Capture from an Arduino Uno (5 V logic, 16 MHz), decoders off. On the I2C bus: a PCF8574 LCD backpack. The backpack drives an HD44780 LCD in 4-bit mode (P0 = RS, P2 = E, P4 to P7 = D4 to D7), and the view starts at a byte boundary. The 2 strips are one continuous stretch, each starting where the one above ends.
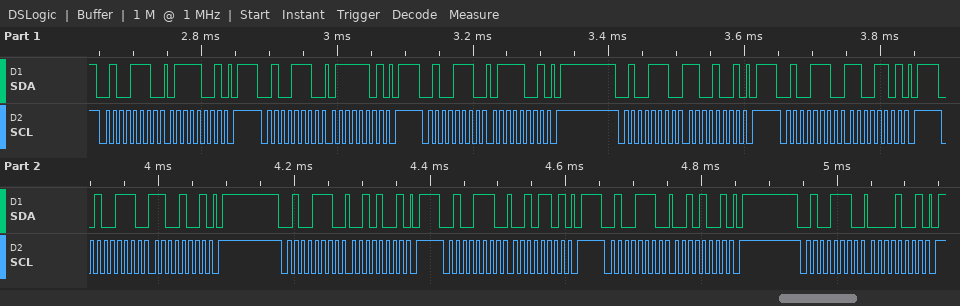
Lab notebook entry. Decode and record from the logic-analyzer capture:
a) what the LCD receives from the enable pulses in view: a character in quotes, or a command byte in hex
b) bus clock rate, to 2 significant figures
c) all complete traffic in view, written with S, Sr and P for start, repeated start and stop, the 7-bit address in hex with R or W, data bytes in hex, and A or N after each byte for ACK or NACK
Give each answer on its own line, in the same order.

'|'
100 kHz
S 27W A 79 A P S 27W A 7D A P S 27W A 79 A P S 27W A C9 A P S 27W A CD A P S 27W A C9 A P S 27W A 29 A P S 27W A 2D A P S 27W A 29 A P S 27W A 09 A P
